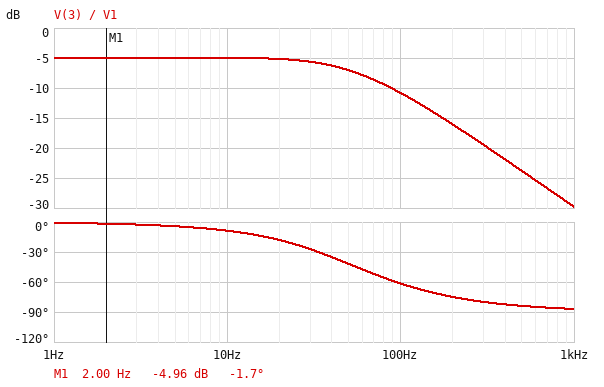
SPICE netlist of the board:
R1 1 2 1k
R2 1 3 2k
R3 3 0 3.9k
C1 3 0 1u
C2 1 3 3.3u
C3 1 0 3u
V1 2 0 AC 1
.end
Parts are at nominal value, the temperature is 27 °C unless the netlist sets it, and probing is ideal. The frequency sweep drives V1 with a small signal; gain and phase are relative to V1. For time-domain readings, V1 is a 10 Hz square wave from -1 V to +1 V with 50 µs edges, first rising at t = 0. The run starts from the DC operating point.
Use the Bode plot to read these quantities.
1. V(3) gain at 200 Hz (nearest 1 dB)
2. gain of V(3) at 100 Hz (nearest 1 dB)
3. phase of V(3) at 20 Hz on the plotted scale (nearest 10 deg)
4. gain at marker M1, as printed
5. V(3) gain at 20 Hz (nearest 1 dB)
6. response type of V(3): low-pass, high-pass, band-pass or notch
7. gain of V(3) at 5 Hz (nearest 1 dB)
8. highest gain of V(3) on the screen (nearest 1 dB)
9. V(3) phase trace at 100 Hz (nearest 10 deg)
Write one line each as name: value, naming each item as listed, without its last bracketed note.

V(3) gain at 200 Hz: -16 dB
gain of V(3) at 100 Hz: -11 dB
phase of V(3) at 20 Hz on the plotted scale: -20 deg
gain at marker M1, as printed: -4.96 dB
V(3) gain at 20 Hz: -5 dB
response type of V(3): low-pass, high-pass, band-pass or notch: low-pass
gain of V(3) at 5 Hz: -5 dB
highest gain of V(3) on the screen: -5 dB
V(3) phase trace at 100 Hz: -60 deg
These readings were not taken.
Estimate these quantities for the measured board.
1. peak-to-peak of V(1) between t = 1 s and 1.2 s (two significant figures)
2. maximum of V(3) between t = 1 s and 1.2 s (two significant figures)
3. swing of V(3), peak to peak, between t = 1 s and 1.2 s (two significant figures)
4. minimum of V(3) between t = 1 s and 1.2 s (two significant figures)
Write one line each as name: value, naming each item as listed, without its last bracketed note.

peak-to-peak of V(1) between t = 1 s and 1.2 s: 1.7 V
maximum of V(3) between t = 1 s and 1.2 s: 580 mV
swing of V(3), peak to peak, between t = 1 s and 1.2 s: 1.2 V
minimum of V(3) between t = 1 s and 1.2 s: -580 mV
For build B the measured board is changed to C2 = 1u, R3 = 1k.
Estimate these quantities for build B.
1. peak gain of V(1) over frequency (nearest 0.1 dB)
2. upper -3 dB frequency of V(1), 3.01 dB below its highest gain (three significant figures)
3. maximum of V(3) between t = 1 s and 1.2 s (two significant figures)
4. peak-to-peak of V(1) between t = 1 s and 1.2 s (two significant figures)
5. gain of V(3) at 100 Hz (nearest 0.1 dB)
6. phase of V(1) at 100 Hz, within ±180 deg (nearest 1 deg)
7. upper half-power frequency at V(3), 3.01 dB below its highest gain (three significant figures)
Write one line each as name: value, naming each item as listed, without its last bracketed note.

peak gain of V(1) over frequency: -2.5 dB
upper -3 dB frequency of V(1), 3.01 dB below its highest gain: 59.5 Hz
maximum of V(3) between t = 1 s and 1.2 s: 250 mV
peak-to-peak of V(1) between t = 1 s and 1.2 s: 1.5 V
gain of V(3) at 100 Hz: -16.0 dB
phase of V(1) at 100 Hz, within ±180 deg: -59 deg
upper half-power frequency at V(3), 3.01 dB below its highest gain: 79.2 Hz
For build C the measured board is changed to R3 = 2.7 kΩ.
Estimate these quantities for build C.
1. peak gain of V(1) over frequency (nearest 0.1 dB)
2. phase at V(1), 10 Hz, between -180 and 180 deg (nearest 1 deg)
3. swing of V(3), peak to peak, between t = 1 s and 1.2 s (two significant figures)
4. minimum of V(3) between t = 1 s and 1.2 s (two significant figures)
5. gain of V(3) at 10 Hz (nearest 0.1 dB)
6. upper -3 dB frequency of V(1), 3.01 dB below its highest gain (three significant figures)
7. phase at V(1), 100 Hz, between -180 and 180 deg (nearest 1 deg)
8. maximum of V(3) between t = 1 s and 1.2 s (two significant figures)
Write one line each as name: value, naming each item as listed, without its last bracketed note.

peak gain of V(1) over frequency: -1.7 dB
phase at V(1), 10 Hz, between -180 and 180 deg: -11 deg
swing of V(3), peak to peak, between t = 1 s and 1.2 s: 1.0 V
minimum of V(3) between t = 1 s and 1.2 s: -510 mV
gain of V(3) at 10 Hz: -6.4 dB
upper -3 dB frequency of V(1), 3.01 dB below its highest gain: 49.6 Hz
phase at V(1), 100 Hz, between -180 and 180 deg: -62 deg
maximum of V(3) between t = 1 s and 1.2 s: 510 mV
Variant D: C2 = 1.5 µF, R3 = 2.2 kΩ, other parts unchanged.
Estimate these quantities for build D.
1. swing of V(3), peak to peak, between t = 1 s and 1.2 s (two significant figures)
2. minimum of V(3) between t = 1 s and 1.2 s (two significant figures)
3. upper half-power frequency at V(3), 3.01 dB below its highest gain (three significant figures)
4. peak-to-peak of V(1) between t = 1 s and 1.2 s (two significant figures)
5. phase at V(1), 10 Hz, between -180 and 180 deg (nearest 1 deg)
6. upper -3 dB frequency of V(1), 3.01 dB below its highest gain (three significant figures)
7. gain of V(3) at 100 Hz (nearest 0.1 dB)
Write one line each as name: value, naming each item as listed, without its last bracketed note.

swing of V(3), peak to peak, between t = 1 s and 1.2 s: 850 mV
minimum of V(3) between t = 1 s and 1.2 s: -420 mV
upper half-power frequency at V(3), 3.01 dB below its highest gain: 62.7 Hz
peak-to-peak of V(1) between t = 1 s and 1.2 s: 1.6 V
phase at V(1), 10 Hz, between -180 and 180 deg: -10 deg
upper -3 dB frequency of V(1), 3.01 dB below its highest gain: 54.5 Hz
gain of V(3) at 100 Hz: -13.0 dB
